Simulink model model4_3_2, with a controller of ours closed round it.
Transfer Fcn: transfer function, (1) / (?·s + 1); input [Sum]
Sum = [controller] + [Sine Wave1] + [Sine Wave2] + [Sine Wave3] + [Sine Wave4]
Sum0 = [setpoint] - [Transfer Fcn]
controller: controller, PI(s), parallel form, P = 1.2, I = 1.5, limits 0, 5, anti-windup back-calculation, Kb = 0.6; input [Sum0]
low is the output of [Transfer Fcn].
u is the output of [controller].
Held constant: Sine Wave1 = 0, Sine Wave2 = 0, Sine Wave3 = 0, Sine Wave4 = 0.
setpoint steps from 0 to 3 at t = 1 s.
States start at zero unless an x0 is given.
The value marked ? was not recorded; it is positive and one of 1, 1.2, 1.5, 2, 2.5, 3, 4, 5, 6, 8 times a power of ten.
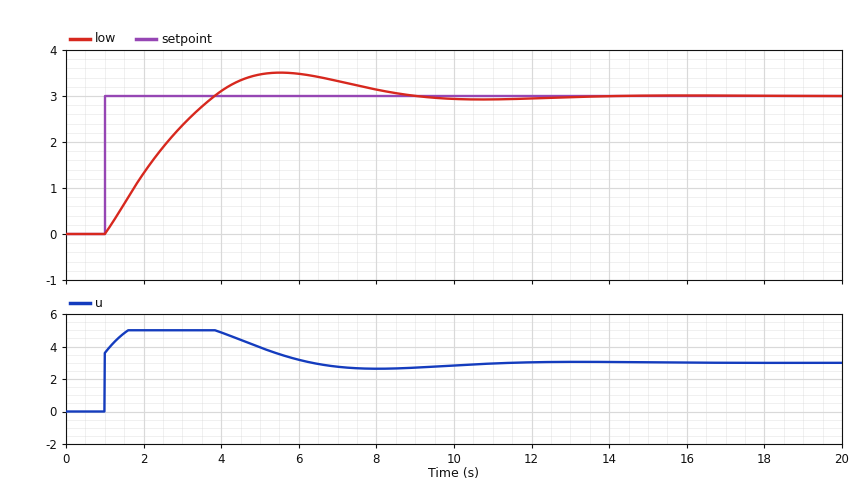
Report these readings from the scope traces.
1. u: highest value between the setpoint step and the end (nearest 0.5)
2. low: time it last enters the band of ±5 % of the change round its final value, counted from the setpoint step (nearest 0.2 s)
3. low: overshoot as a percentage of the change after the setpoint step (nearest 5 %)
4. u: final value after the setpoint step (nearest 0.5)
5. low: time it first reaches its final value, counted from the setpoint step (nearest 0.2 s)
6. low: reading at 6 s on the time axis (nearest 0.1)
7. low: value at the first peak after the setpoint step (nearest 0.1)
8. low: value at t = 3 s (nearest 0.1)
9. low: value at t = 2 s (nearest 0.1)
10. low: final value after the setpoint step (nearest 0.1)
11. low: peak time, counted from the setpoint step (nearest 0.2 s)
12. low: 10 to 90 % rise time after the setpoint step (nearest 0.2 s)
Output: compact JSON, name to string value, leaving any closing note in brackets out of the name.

{"u: highest value between the setpoint step and the end": "5.0", "low: time it last enters the band of ±5 % of the change round its final value, counted from the setpoint step": "7.0 s", "low: overshoot as a percentage of the change after the setpoint step": "15 %", "u: final value after the setpoint step": "3.0", "low: time it first reaches its final value, counted from the setpoint step": "2.8 s", "low: reading at 6 s on the time axis": "3.5", "low: value at the first peak after the setpoint step": "3.5", "low: value at t = 3 s": "2.4", "low: value at t = 2 s": "1.3", "low: final value after the setpoint step": "3.0", "low: peak time, counted from the setpoint step": "4.6 s", "low: 10 to 90 % rise time after the setpoint step": "2.2 s"}
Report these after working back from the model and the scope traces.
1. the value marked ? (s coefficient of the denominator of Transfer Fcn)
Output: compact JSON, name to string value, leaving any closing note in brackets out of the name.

{"the value marked ?": "3"}
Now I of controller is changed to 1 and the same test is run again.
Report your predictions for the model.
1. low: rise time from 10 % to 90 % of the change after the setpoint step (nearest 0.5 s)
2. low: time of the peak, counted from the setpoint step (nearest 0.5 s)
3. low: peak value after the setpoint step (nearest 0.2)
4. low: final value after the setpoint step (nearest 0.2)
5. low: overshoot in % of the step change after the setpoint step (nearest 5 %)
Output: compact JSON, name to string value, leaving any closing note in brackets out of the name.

{"low: rise time from 10 % to 90 % of the change after the setpoint step": "2.5 s", "low: time of the peak, counted from the setpoint step": "5.5 s", "low: peak value after the setpoint step": "3.4", "low: final value after the setpoint step": "3.0", "low: overshoot in % of the step change after the setpoint step": "10 %"}
